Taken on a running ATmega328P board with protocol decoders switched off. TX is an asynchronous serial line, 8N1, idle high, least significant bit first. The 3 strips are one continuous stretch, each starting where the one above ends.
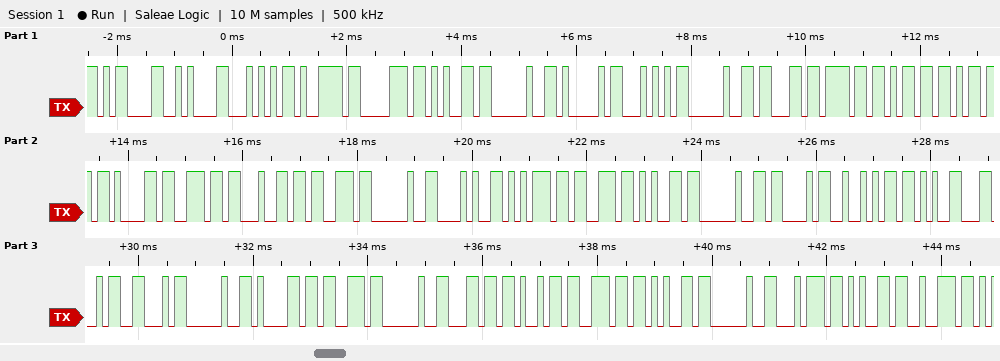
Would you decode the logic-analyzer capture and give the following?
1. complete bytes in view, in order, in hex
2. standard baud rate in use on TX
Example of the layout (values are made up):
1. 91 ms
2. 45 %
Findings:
1. 0D 0A 54 79 70 65 20 41 54 20 63 6F 6D 6D 61 6E 64 73 20 28 75 73 65 20 43 52 2B 4C 46 20 61 73 20 6C 69 6E 65 20 74 65 72
2. 9600 baud
